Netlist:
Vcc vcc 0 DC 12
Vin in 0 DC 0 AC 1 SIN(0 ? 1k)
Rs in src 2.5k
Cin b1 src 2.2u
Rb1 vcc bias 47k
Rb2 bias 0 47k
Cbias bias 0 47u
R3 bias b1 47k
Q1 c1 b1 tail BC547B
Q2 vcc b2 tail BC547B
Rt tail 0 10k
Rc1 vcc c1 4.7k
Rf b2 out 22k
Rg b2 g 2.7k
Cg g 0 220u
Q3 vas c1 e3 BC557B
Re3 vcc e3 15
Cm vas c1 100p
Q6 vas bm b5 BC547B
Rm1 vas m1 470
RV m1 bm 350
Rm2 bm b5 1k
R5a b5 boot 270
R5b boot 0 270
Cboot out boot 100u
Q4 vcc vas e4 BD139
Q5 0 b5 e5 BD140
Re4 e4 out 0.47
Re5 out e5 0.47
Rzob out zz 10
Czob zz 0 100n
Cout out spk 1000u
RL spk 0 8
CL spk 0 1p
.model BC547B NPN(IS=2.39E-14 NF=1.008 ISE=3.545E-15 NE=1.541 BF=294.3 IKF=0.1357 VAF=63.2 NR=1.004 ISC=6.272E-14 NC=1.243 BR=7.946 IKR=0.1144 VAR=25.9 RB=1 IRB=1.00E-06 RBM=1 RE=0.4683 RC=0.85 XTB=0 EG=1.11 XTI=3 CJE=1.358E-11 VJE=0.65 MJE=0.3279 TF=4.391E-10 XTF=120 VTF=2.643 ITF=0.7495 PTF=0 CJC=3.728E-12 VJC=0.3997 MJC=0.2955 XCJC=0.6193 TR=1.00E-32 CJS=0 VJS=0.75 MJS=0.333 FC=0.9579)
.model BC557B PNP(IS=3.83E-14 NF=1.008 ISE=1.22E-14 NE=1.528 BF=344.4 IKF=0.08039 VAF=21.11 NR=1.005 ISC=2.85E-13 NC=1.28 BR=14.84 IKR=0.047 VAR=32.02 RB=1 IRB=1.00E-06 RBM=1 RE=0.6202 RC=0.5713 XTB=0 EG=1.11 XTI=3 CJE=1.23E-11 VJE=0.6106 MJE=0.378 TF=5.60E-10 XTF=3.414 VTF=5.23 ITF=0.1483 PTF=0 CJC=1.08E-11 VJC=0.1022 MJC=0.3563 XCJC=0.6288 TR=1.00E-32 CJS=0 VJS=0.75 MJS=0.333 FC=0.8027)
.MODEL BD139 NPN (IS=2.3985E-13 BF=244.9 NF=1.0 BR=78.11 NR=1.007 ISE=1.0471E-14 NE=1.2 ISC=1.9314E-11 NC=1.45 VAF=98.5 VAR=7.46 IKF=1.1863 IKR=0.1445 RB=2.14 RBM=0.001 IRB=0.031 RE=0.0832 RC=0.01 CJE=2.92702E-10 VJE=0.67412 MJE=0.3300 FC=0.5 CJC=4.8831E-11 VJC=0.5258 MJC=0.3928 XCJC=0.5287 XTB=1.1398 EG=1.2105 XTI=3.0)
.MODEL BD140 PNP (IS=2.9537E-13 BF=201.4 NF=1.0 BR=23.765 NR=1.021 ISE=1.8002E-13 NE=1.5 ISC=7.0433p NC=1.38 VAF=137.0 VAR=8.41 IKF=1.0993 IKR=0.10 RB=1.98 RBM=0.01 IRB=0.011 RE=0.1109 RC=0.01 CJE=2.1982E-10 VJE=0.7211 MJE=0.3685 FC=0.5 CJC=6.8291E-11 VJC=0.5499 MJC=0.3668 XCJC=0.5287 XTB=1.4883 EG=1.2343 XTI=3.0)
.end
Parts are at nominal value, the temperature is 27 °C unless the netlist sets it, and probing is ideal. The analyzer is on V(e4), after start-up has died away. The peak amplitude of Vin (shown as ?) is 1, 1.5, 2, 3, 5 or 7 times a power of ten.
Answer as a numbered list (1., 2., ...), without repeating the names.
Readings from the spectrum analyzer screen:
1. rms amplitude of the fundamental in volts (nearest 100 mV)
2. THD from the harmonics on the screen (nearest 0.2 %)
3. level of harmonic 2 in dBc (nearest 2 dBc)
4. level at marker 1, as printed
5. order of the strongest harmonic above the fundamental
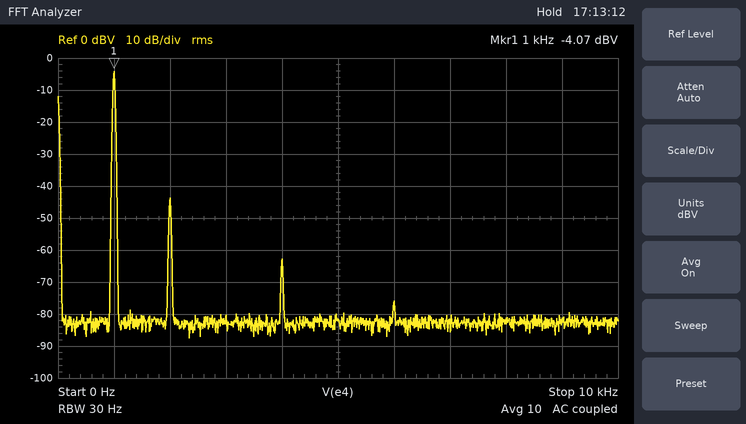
1. 600 mV
2. 1.0 %
3. -40 dBc
4. -4.07 dBV
5. 2
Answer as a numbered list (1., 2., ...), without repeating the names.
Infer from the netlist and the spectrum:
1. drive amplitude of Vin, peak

1. 100 mV
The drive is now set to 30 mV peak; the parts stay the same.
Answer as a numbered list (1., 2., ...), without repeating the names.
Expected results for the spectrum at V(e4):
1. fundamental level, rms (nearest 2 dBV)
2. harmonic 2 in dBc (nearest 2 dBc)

1. -14 dBV
2. -46 dBc
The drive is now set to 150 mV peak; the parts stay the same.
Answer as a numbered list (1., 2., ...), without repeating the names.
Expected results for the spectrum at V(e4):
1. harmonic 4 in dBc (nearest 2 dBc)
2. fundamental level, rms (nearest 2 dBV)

1. -56 dBc
2. 0 dBV
